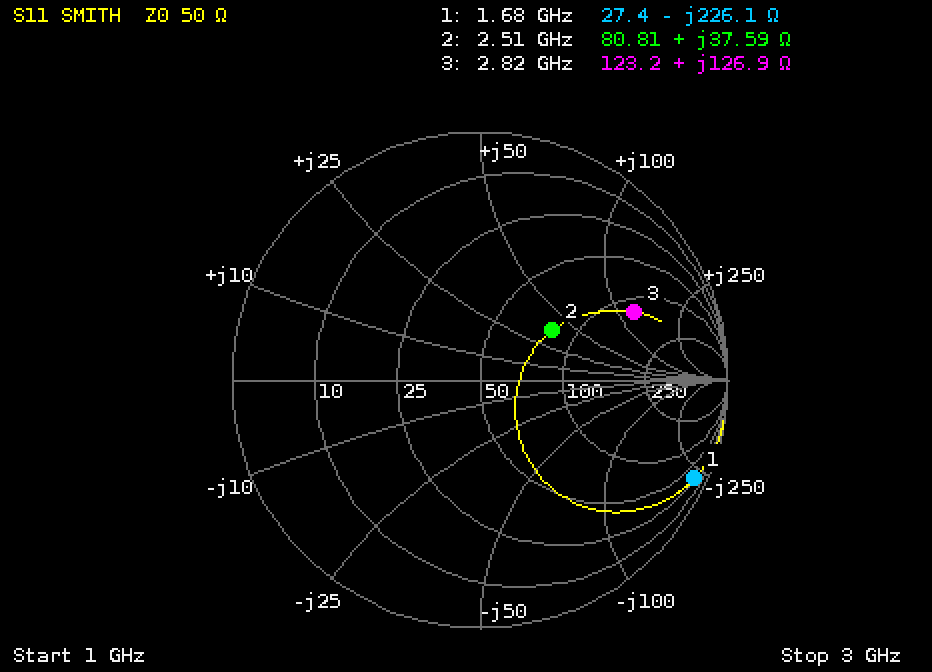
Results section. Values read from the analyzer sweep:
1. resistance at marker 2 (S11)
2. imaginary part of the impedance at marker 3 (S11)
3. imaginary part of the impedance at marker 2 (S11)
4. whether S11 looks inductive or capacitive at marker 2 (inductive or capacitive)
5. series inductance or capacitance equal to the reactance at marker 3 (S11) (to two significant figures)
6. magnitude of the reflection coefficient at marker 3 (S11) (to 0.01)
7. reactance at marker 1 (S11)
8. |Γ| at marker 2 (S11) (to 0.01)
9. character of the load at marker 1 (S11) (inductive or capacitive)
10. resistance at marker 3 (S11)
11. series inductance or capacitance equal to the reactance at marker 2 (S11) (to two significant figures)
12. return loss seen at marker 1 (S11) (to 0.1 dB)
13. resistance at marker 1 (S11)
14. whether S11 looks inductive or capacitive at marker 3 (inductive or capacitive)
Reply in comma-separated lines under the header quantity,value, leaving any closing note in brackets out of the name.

quantity,value
resistance at marker 2,80.81 Ω
imaginary part of the impedance at marker 3,+126.9 Ω
imaginary part of the impedance at marker 2,+37.59 Ω
whether S11 looks inductive or capacitive at marker 2,inductive
series inductance or capacitance equal to the reactance at marker 3 (S11),7.2 nH
magnitude of the reflection coefficient at marker 3 (S11),0.68
reactance at marker 1,-226.1 Ω
|Γ| at marker 2 (S11),0.36
character of the load at marker 1 (S11),capacitive
resistance at marker 3,123.2 Ω
series inductance or capacitance equal to the reactance at marker 2 (S11),2.4 nH
return loss seen at marker 1 (S11),0.4 dB
resistance at marker 1,27.4 Ω
whether S11 looks inductive or capacitive at marker 3,inductive
